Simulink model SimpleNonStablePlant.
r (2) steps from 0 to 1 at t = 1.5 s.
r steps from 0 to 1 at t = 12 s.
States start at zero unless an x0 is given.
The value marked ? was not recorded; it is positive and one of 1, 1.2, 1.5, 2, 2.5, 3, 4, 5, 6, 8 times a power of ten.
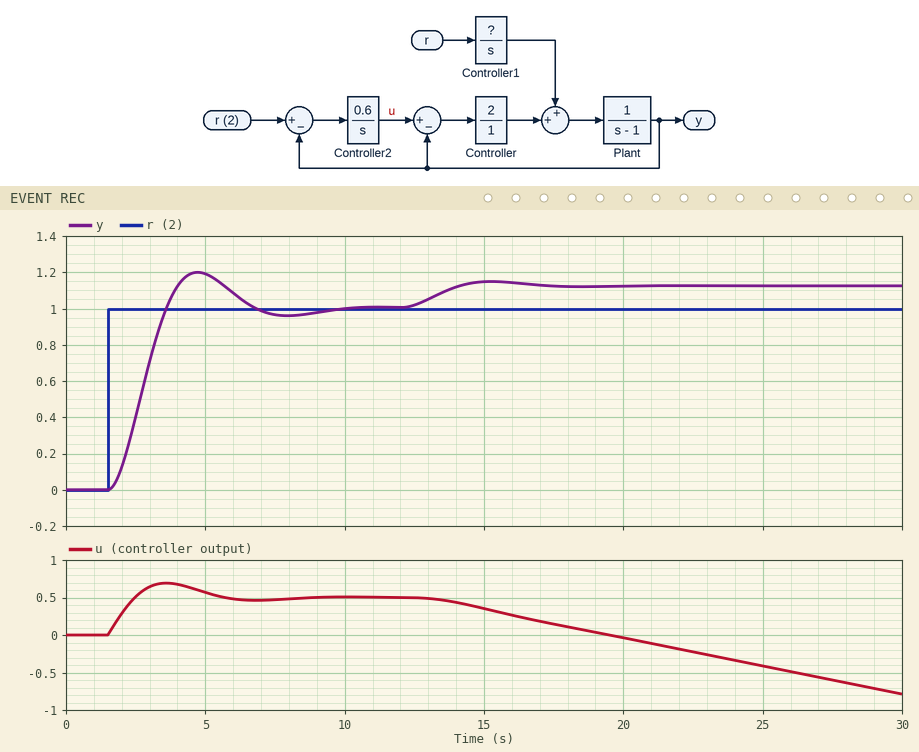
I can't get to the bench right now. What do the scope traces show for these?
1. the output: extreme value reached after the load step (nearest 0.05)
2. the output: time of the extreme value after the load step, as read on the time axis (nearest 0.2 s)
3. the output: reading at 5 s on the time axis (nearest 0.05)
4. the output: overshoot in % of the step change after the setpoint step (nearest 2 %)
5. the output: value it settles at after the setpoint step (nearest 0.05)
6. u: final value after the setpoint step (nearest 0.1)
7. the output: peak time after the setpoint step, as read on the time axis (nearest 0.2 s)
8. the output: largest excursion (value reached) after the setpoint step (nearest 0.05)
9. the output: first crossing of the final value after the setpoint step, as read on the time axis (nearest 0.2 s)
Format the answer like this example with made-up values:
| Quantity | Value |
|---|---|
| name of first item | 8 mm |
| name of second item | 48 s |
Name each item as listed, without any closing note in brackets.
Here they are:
| Quantity | Value |
|---|---|
| the output: extreme value reached after the load step | 1.15 |
| the output: time of the extreme value after the load step, as read on the time axis | 15.2 s |
| the output: reading at 5 s on the time axis | 1.20 |
| the output: overshoot in % of the step change after the setpoint step | 20 % |
| the output: value it settles at after the setpoint step | 1.00 |
| u: final value after the setpoint step | 0.5 |
| the output: peak time after the setpoint step, as read on the time axis | 4.8 s |
| the output: largest excursion (value reached) after the setpoint step | 1.20 |
| the output: first crossing of the final value after the setpoint step, as read on the time axis | 3.6 s |
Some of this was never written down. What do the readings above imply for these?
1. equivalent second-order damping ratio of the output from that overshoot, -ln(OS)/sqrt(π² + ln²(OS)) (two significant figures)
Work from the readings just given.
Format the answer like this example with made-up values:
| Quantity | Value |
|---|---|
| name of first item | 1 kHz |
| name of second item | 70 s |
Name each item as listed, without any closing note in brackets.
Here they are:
| Quantity | Value |
|---|---|
| equivalent second-order damping ratio of the output from that overshoot, -ln(OS)/sqrt(π² + ln²(OS)) | 0.46 |
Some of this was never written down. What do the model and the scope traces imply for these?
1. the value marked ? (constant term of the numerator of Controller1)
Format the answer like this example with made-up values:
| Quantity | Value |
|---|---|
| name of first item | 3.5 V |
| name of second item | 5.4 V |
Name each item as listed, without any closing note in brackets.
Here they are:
| Quantity | Value |
|---|---|
| the value marked ? | 0.15 |
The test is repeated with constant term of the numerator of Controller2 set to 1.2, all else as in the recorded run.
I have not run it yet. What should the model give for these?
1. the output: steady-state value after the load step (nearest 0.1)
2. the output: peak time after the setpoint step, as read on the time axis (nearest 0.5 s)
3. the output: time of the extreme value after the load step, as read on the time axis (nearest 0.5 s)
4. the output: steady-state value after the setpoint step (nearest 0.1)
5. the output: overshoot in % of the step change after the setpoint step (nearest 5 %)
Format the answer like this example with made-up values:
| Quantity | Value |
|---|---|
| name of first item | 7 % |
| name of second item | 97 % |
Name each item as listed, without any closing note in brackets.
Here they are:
| Quantity | Value |
|---|---|
| the output: steady-state value after the load step | 1.1 |
| the output: peak time after the setpoint step, as read on the time axis | 3.5 s |
| the output: time of the extreme value after the load step, as read on the time axis | 14.0 s |
| the output: steady-state value after the setpoint step | 1.0 |
| the output: overshoot in % of the step change after the setpoint step | 35 % |
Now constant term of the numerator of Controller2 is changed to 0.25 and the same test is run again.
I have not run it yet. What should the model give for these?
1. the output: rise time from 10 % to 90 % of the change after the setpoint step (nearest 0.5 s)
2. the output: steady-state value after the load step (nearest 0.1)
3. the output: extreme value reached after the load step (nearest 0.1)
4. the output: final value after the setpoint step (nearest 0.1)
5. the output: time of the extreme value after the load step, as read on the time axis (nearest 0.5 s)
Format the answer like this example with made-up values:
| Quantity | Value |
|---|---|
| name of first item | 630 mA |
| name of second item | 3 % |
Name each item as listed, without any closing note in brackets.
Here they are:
| Quantity | Value |
|---|---|
| the output: rise time from 10 % to 90 % of the change after the setpoint step | 3.0 s |
| the output: steady-state value after the load step | 1.3 |
| the output: extreme value reached after the load step | 1.3 |
| the output: final value after the setpoint step | 1.0 |
| the output: time of the extreme value after the load step, as read on the time axis | 18.5 s |
